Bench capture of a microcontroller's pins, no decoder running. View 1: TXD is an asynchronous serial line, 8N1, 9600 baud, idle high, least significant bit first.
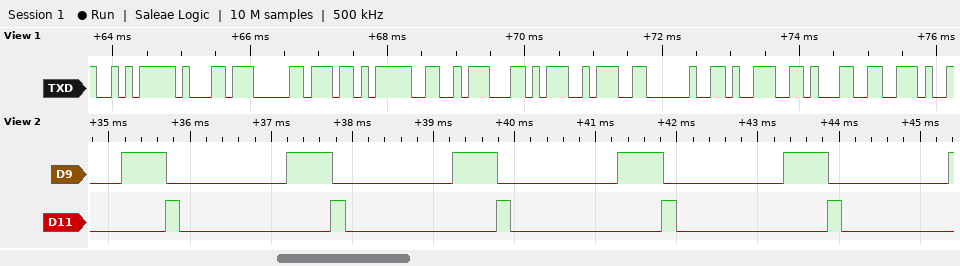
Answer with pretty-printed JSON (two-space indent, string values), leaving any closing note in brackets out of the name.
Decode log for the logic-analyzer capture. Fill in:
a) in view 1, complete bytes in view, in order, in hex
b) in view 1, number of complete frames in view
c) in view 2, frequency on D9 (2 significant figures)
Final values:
{
  "in view 1, complete bytes in view, in order, in hex": "EA B1 B0 EB A6 AC 3A 20 39 31 2E",
  "in view 1, number of complete frames in view": "11",
  "in view 2, frequency on D9": "490 Hz"
}
